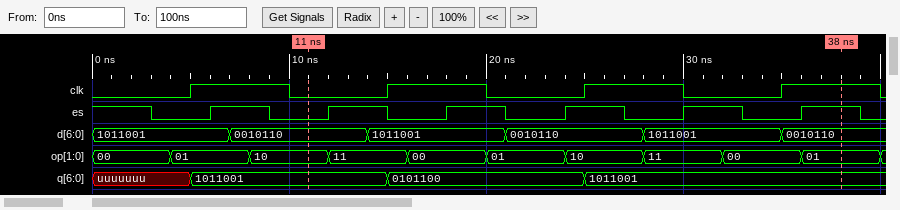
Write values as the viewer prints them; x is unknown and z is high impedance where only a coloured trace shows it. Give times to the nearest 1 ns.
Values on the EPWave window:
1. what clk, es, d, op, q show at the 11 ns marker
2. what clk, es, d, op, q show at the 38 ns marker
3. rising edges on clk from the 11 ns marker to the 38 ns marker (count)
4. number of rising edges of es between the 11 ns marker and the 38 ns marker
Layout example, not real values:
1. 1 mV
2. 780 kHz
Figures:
1. clk=0, es=0, d=0010110, op=10, q=1011001
2. clk=1, es=1, d=0010110, op=01, q=1011001
3. 3
4. 5
